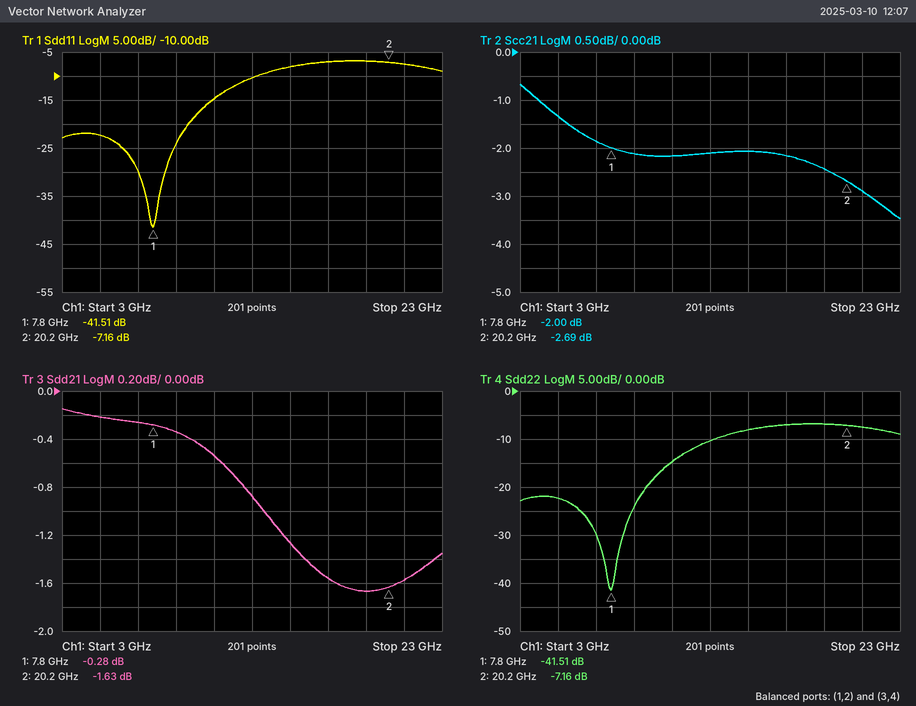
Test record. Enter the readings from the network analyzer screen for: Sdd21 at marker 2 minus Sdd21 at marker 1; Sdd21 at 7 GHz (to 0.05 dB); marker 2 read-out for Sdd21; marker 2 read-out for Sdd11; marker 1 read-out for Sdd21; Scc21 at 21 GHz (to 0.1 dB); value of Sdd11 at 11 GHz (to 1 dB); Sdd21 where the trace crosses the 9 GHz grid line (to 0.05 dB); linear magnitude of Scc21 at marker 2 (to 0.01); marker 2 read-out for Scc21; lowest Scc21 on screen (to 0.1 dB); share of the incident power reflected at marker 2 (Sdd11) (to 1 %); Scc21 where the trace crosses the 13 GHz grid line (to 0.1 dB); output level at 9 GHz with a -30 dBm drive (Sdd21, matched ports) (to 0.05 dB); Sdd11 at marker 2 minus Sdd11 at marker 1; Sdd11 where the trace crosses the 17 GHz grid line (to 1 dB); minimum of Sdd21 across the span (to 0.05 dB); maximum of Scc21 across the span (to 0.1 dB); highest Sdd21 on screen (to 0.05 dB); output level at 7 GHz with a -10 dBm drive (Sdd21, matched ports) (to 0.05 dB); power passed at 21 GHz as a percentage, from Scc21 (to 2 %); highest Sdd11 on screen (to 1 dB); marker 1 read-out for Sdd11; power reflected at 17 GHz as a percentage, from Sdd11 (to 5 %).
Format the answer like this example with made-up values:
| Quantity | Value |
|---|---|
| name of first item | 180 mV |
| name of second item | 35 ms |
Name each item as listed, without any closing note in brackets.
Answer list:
| Quantity | Value |
|---|---|
| Sdd21 at marker 2 minus Sdd21 at marker 1 | -1.35 dB |
| Sdd21 at 7 GHz | -0.25 dB |
| marker 2 read-out for Sdd21 | -1.63 dB |
| marker 2 read-out for Sdd11 | -7.16 dB |
| marker 1 read-out for Sdd21 | -0.28 dB |
| Scc21 at 21 GHz | -2.9 dB |
| value of Sdd11 at 11 GHz | -15 dB |
| Sdd21 where the trace crosses the 9 GHz grid line | -0.35 dB |
| linear magnitude of Scc21 at marker 2 | 0.73 |
| marker 2 read-out for Scc21 | -2.69 dB |
| lowest Scc21 on screen | -3.5 dB |
| share of the incident power reflected at marker 2 (Sdd11) | 19 % |
| Scc21 where the trace crosses the 13 GHz grid line | -2.1 dB |
| output level at 9 GHz with a -30 dBm drive (Sdd21, matched ports) | -30.35 dBm |
| Sdd11 at marker 2 minus Sdd11 at marker 1 | 34.35 dB |
| Sdd11 where the trace crosses the 17 GHz grid line | -7 dB |
| minimum of Sdd21 across the span | -1.65 dB |
| maximum of Scc21 across the span | -0.7 dB |
| highest Sdd21 on screen | -0.15 dB |
| output level at 7 GHz with a -10 dBm drive (Sdd21, matched ports) | -10.25 dBm |
| power passed at 21 GHz as a percentage, from Scc21 | 52 % |
| highest Sdd11 on screen | -7 dB |
| marker 1 read-out for Sdd11 | -41.51 dB |
| power reflected at 17 GHz as a percentage, from Sdd11 | 20 % |
